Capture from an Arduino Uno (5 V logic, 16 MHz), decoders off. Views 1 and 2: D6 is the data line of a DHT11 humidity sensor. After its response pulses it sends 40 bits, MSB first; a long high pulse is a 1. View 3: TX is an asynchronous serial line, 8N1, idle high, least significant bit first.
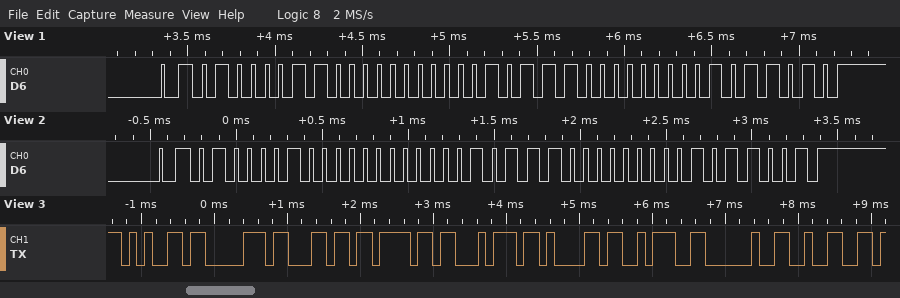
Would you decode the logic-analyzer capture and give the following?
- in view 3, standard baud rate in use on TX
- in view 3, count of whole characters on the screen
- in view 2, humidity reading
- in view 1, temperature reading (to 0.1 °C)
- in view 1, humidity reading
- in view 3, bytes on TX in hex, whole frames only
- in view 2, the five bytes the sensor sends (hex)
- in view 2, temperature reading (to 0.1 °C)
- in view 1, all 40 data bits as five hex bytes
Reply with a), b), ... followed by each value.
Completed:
a) 9600 baud
b) 9
c) 66 %
d) 23.0 °C
e) 67 %
f) 65 70 6C 6F 74 61 3A 20 32
g) 42 00 17 00 59
h) 23.0 °C
i) 43 00 17 00 5A
